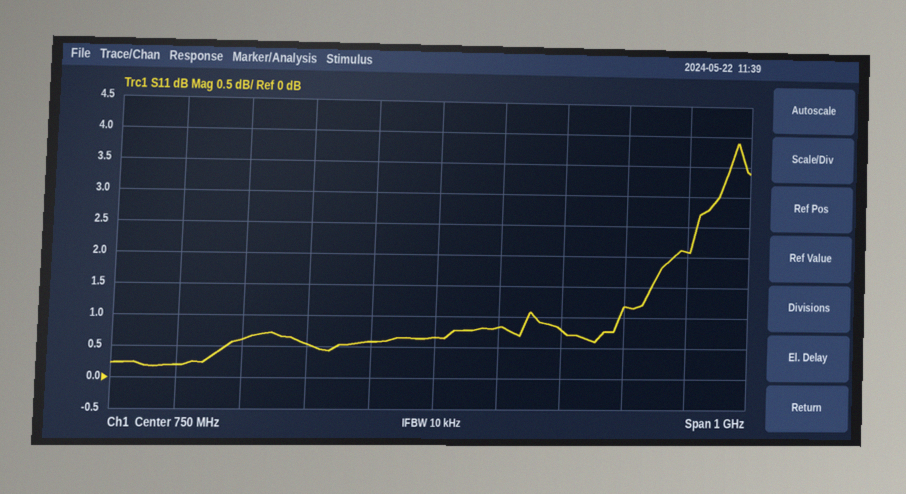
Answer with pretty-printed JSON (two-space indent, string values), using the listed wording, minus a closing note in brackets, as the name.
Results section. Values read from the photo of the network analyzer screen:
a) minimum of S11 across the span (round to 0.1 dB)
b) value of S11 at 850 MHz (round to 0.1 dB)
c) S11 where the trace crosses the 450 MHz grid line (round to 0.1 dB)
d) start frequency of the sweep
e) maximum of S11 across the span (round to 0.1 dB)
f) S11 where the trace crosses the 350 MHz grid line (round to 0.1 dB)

{
  "minimum of S11 across the span": "0.2 dB",
  "value of S11 at 850 MHz": "0.8 dB",
  "S11 where the trace crosses the 450 MHz grid line": "0.6 dB",
  "start frequency of the sweep": "250 MHz",
  "maximum of S11 across the span": "3.9 dB",
  "S11 where the trace crosses the 350 MHz grid line": "0.2 dB"
}
